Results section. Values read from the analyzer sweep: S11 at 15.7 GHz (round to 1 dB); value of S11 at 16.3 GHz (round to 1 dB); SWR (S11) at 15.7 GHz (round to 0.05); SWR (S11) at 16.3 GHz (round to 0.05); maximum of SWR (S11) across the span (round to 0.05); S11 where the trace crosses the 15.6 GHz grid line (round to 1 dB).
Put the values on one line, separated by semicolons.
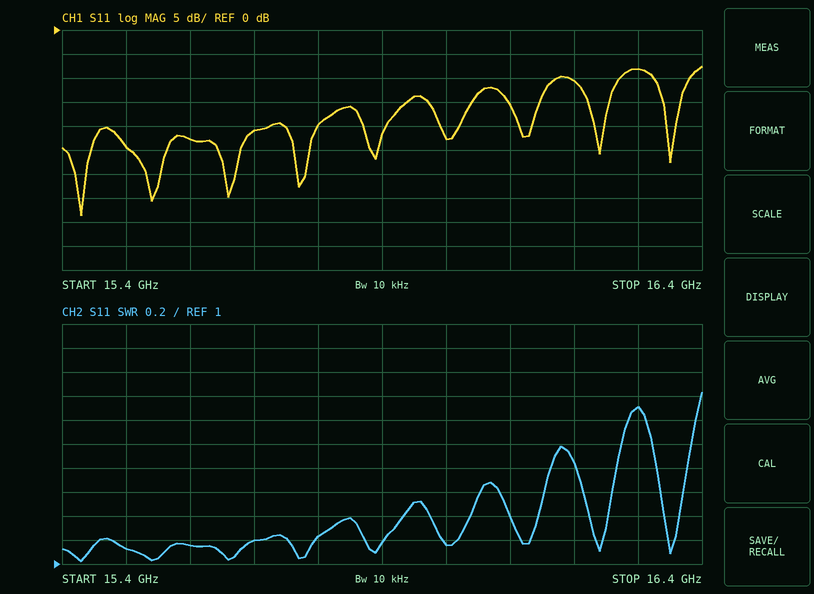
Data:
-21 dB; -8 dB; 1.20; 2.30; 2.45; -23 dB
